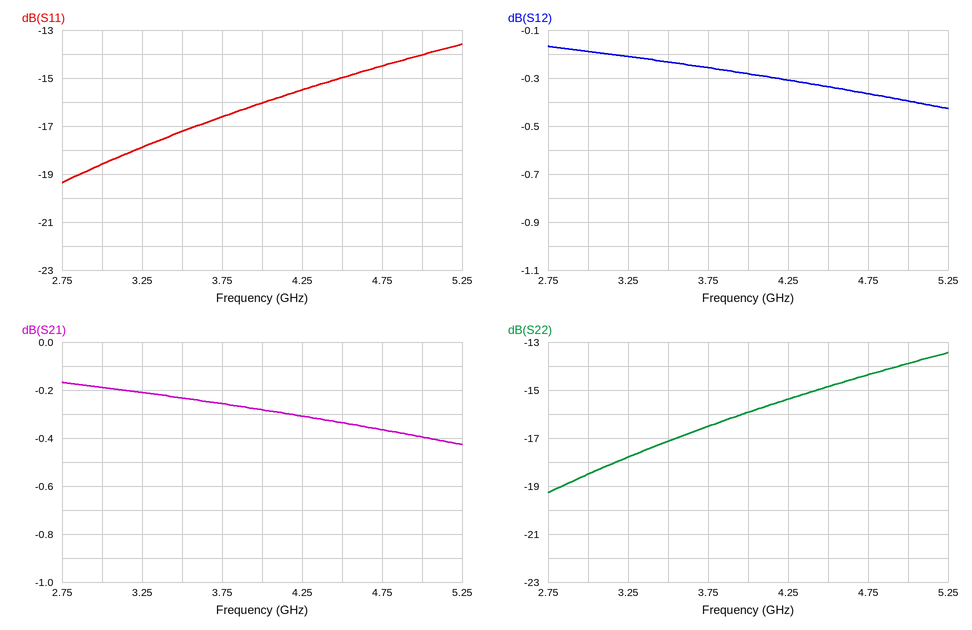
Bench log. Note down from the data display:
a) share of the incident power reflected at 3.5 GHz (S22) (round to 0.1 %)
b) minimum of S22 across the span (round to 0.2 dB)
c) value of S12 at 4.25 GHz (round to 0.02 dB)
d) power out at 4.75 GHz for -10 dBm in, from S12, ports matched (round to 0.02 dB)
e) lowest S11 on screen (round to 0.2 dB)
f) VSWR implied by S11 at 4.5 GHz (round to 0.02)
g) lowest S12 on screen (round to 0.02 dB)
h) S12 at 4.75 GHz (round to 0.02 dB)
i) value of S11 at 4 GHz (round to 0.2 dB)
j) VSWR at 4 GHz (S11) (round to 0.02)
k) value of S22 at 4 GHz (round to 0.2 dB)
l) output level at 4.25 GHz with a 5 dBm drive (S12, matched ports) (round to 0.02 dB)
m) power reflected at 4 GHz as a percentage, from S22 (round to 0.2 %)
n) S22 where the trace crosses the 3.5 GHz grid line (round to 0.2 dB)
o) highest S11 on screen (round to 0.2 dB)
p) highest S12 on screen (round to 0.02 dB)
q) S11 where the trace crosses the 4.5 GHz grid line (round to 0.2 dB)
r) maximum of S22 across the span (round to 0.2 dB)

1.9 %
-19.2 dB
-0.30 dB
-10.36 dBm
-19.4 dB
1.44
-0.42 dB
-0.36 dB
-16.0 dB
1.38
-16.0 dB
4.70 dBm
2.6 %
-17.2 dB
-13.6 dB
-0.16 dB
-15.0 dB
-13.4 dB
